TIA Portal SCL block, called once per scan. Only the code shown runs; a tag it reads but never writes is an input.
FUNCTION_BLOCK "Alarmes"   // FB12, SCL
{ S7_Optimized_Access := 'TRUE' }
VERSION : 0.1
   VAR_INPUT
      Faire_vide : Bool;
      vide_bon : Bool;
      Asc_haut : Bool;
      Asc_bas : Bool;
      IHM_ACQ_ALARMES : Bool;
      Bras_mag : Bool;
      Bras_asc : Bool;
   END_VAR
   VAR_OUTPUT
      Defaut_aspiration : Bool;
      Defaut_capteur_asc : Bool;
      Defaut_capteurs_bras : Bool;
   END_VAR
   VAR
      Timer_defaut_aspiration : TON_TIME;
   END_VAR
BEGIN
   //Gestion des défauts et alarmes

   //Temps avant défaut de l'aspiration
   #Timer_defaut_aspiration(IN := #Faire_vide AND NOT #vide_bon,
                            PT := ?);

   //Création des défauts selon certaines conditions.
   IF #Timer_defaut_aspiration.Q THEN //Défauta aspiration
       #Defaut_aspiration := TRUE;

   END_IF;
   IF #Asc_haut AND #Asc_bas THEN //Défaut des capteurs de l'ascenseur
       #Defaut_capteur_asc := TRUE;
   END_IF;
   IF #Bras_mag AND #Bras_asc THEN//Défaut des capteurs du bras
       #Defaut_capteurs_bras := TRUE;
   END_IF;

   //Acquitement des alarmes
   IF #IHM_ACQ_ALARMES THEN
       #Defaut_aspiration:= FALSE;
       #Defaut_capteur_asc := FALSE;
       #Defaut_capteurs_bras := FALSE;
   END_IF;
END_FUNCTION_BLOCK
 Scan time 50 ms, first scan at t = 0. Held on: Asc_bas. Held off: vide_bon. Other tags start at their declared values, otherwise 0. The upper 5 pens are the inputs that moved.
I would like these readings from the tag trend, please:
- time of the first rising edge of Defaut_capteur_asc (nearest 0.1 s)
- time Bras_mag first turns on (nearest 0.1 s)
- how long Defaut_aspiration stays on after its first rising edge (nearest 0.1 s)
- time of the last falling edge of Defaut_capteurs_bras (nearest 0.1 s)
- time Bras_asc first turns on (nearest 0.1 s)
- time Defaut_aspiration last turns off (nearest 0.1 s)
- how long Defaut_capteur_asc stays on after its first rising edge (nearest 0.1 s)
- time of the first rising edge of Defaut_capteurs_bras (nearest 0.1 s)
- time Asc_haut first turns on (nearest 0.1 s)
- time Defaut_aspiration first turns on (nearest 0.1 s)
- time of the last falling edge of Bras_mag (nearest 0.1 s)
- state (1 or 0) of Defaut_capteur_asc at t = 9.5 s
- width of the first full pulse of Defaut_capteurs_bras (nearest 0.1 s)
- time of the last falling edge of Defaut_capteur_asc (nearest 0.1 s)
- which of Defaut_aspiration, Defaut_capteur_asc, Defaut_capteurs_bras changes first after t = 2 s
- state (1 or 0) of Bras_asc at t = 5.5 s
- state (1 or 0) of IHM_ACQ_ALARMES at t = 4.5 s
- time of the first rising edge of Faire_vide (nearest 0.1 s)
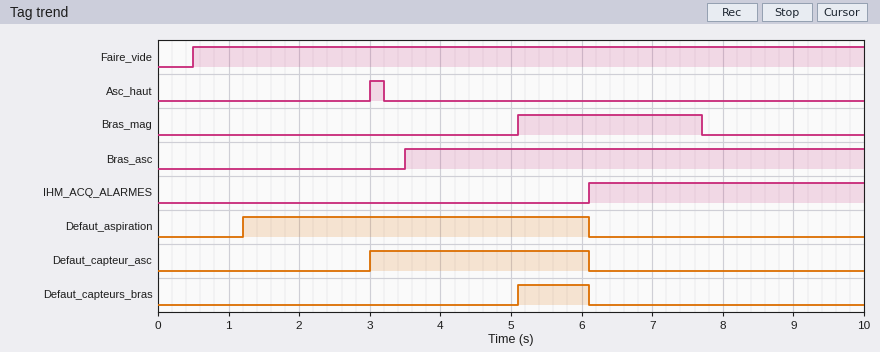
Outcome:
3.0 s
5.1 s
4.9 s
6.1 s
3.5 s
6.1 s
3.1 s
5.1 s
3.0 s
1.2 s
7.7 s
0
1.0 s
6.1 s
Defaut_capteur_asc
1
0
0.5 s
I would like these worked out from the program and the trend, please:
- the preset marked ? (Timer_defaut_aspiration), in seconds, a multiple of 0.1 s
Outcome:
0.7 s
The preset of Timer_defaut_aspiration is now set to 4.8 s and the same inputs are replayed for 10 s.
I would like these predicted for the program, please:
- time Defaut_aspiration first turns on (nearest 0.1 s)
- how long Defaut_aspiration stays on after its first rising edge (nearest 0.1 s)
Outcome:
5.3 s
0.8 s
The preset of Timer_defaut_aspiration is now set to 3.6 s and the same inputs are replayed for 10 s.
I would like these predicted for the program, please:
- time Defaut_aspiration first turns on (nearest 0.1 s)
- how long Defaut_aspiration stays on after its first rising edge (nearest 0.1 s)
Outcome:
4.1 s
2.0 s
